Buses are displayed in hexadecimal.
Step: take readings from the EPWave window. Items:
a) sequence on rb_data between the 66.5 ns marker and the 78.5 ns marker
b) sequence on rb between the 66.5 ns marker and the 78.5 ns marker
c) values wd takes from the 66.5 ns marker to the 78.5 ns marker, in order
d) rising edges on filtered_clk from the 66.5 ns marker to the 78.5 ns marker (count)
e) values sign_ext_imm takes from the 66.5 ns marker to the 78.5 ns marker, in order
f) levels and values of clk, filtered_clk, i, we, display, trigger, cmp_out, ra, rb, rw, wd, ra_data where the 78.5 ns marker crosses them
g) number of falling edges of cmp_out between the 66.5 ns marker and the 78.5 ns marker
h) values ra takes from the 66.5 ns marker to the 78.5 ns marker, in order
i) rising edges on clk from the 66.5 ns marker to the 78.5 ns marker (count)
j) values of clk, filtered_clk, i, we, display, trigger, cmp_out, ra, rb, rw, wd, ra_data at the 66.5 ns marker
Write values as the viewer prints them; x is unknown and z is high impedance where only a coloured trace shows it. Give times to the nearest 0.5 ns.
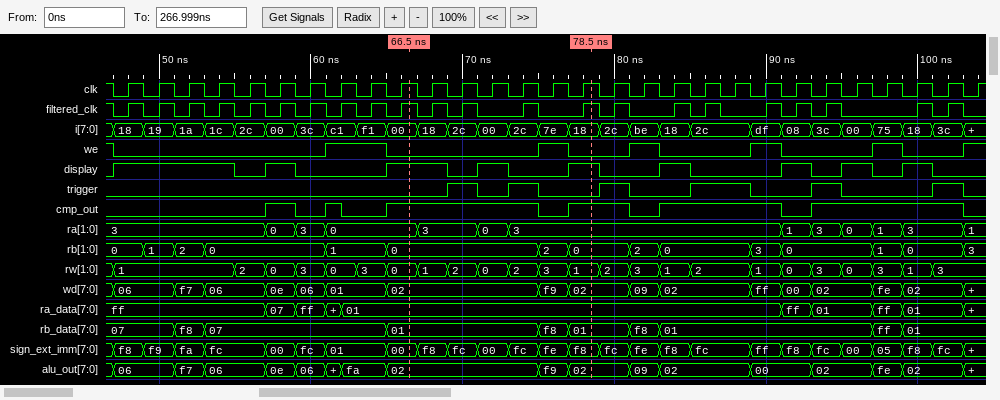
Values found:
01, f8, 01
0, 2, 0
02, f9, 02
4
00, f8, fc, 00, fc, fe, f8
clk=1, filtered_clk=1, i=18, we=0, display=1, trigger=0, cmp_out=1, ra=3, rb=0, rw=1, wd=02, ra_data=01
1
0, 3, 0, 3
6
clk=1, filtered_clk=1, i=00, we=0, display=1, trigger=0, cmp_out=1, ra=0, rb=0, rw=0, wd=02, ra_data=01
